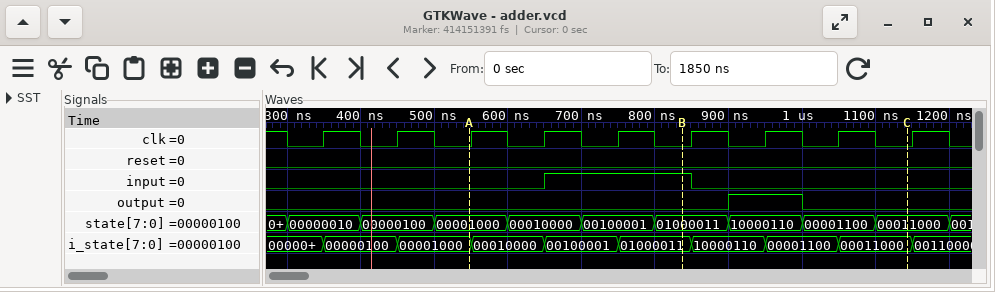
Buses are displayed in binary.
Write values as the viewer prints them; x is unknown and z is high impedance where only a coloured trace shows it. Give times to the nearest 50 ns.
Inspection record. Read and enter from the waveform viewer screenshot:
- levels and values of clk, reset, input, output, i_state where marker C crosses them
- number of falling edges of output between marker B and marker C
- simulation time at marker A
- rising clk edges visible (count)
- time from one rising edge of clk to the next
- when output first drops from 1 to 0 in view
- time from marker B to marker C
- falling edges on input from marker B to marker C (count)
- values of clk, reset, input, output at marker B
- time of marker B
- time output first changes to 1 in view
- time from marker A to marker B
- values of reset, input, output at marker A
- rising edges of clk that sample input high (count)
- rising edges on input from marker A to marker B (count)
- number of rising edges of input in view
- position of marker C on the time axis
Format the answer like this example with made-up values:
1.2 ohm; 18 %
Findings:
clk=0, reset=0, input=0, output=0, i_state=00011000; 1; 550 ns; 9; 100 ns; 1000 ns; 300 ns; 1; clk=0, reset=0, input=1, output=0; 850 ns; 900 ns; 300 ns; reset=0, input=0, output=0; 2; 1; 1; 1150 ns
